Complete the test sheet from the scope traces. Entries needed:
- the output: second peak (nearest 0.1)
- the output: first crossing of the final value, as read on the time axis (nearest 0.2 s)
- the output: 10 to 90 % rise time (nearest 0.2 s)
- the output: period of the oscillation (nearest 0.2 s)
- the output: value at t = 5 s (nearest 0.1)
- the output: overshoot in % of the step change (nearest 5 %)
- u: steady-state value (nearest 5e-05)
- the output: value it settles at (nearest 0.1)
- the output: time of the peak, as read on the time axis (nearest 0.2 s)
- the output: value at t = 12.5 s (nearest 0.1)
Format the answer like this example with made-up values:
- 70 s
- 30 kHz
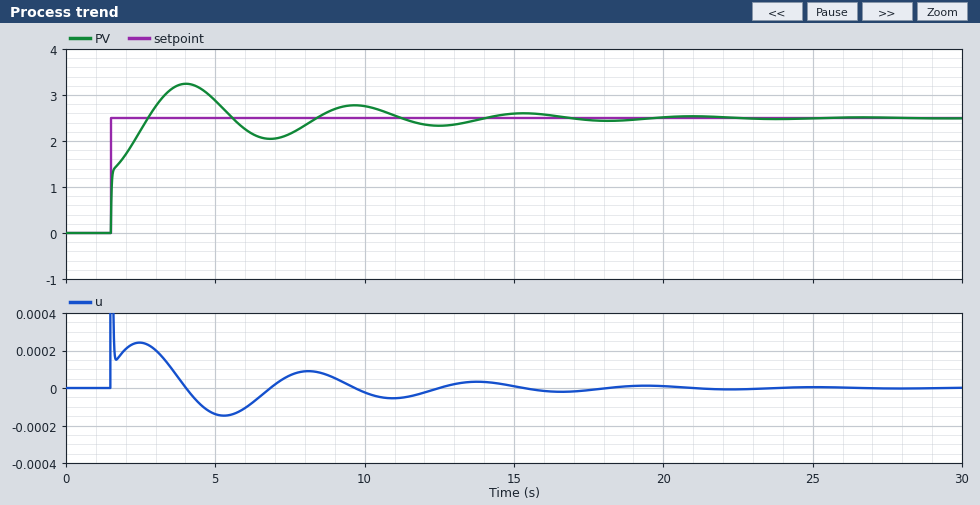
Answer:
- 2.8
- 2.8 s
- 1.0 s
- 5.6 s
- 2.9
- 30 %
- 0.00000
- 2.5
- 4.0 s
- 2.3
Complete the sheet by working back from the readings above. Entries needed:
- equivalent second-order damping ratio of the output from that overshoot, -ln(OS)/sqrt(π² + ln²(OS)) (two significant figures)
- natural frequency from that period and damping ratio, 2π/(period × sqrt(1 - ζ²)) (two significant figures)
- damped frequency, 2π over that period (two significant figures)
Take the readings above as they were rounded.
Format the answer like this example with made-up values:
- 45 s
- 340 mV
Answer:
- 0.36
- 1.2 rad/s
- 1.1 rad/s
